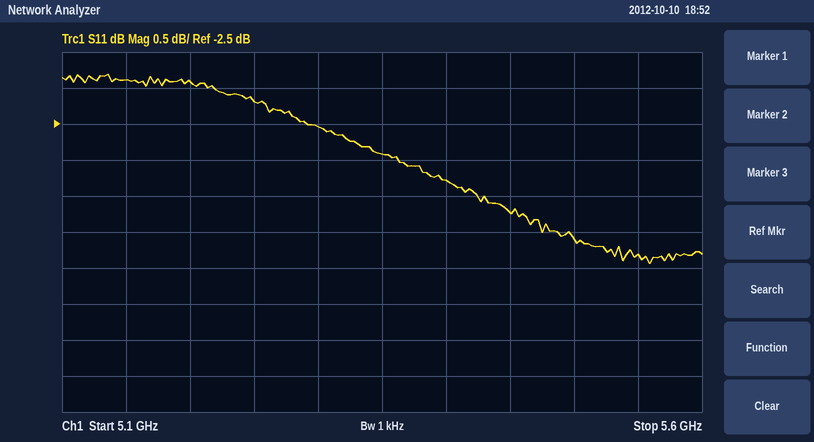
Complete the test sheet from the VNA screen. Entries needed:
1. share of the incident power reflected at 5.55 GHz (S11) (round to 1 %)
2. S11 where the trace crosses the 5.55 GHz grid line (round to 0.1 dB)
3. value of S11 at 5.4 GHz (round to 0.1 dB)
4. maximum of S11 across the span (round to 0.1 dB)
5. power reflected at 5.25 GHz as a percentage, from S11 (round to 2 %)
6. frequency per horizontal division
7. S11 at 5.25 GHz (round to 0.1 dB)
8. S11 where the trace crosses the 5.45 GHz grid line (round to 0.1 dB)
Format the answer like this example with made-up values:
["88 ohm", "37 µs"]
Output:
["37 %", "-4.3 dB", "-3.3 dB", "-1.8 dB", "60 %", "50 MHz", "-2.2 dB", "-3.7 dB"]
